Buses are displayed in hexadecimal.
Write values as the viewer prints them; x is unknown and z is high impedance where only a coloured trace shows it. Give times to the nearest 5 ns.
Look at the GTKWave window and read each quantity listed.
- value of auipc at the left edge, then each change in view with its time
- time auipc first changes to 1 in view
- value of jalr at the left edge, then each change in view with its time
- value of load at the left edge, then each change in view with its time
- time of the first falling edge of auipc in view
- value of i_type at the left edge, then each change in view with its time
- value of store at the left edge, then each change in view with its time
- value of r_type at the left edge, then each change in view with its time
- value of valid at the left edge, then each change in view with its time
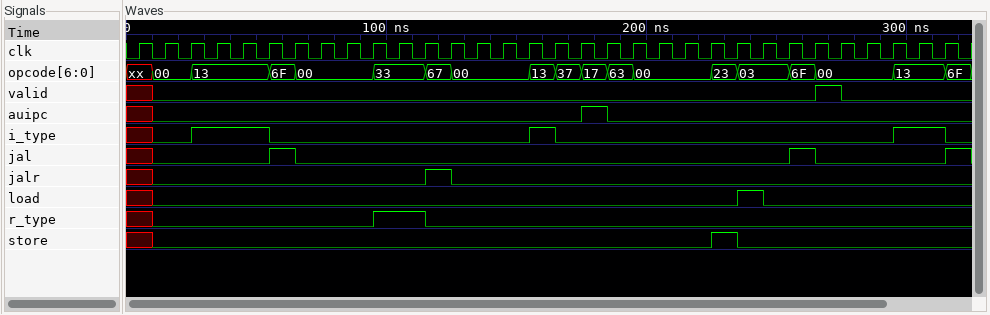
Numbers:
x, 0 at 10 ns, 1 at 175 ns, 0 at 185 ns
175 ns
x, 0 at 10 ns, 1 at 115 ns, 0 at 125 ns
x, 0 at 10 ns, 1 at 235 ns, 0 at 245 ns
185 ns
x, 0 at 10 ns, 1 at 25 ns, 0 at 55 ns, 1 at 155 ns, 0 at 165 ns, 1 at 295 ns, 0 at 315 ns
x, 0 at 10 ns, 1 at 225 ns, 0 at 235 ns
x, 0 at 10 ns, 1 at 95 ns, 0 at 115 ns
x, 0 at 10 ns, 1 at 265 ns, 0 at 275 ns
